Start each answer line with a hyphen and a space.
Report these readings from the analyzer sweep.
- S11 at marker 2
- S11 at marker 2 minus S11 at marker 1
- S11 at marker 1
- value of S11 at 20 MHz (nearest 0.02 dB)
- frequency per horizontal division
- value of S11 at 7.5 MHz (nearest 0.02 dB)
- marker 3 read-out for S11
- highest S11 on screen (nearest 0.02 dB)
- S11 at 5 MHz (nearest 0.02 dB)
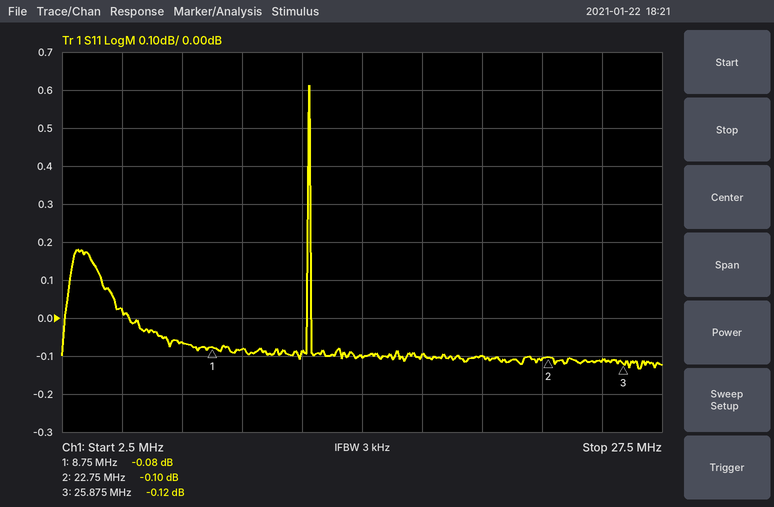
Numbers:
- -0.10 dB
- -0.02 dB
- -0.08 dB
- -0.10 dB
- 2.5 MHz
- -0.06 dB
- -0.12 dB
- 0.62 dB
- 0.02 dB
